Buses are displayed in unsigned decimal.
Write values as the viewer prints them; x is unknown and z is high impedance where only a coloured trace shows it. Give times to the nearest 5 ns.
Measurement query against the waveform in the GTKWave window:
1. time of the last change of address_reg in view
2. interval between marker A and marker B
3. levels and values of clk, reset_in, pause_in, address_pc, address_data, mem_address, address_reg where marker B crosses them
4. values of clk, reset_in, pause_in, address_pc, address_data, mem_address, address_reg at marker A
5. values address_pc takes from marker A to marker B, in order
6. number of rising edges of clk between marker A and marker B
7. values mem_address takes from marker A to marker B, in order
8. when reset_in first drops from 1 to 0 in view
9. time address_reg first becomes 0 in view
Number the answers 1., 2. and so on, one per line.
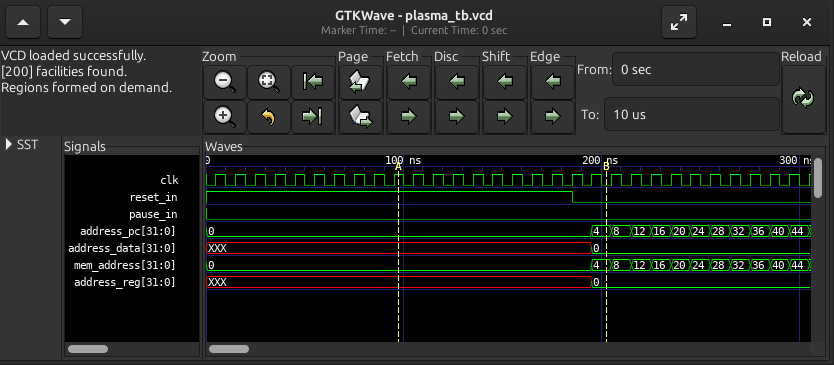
1. 195 ns
2. 105 ns
3. clk=0, reset_in=0, pause_in=0, address_pc=4, address_data=0, mem_address=4, address_reg=0
4. clk=1, reset_in=1, pause_in=0, address_pc=0, address_data=XXX, mem_address=0, address_reg=XXX
5. 0, 4
6. 10
7. 0, 4
8. 185 ns
9. 195 ns
